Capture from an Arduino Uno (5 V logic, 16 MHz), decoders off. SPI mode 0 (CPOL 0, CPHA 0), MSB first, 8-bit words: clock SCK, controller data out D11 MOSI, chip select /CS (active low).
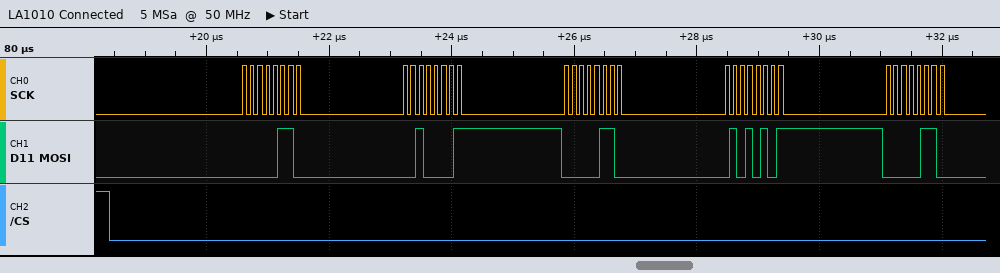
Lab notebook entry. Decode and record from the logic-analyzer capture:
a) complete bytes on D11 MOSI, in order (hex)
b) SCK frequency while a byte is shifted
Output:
06 21 06 55 06
8 MHz
